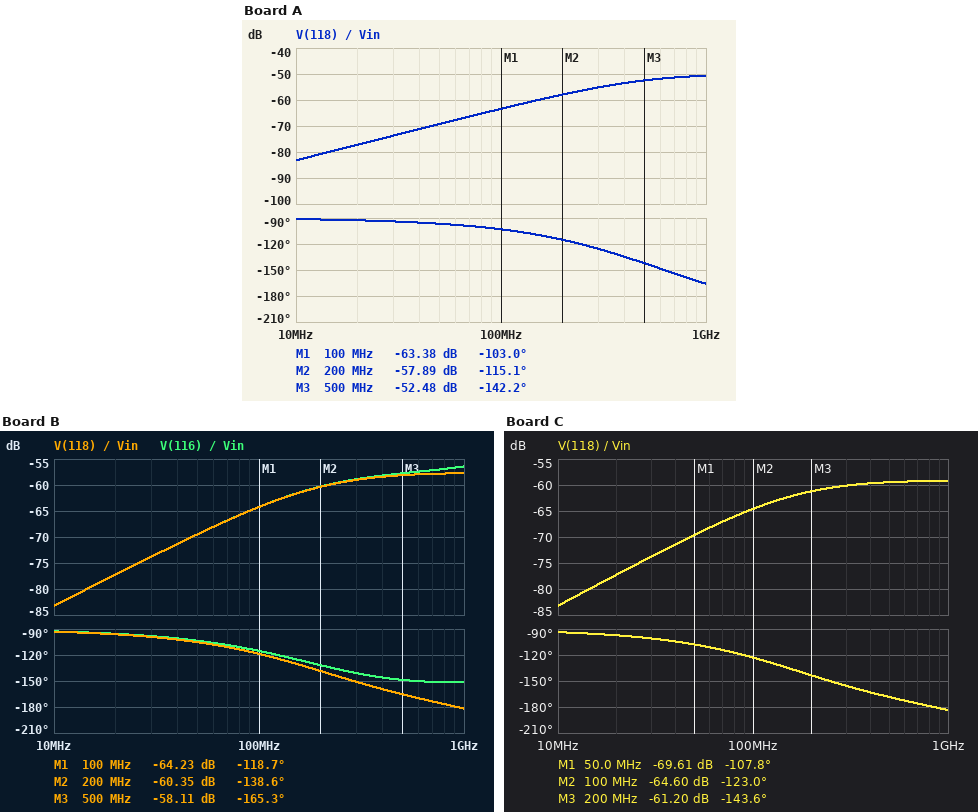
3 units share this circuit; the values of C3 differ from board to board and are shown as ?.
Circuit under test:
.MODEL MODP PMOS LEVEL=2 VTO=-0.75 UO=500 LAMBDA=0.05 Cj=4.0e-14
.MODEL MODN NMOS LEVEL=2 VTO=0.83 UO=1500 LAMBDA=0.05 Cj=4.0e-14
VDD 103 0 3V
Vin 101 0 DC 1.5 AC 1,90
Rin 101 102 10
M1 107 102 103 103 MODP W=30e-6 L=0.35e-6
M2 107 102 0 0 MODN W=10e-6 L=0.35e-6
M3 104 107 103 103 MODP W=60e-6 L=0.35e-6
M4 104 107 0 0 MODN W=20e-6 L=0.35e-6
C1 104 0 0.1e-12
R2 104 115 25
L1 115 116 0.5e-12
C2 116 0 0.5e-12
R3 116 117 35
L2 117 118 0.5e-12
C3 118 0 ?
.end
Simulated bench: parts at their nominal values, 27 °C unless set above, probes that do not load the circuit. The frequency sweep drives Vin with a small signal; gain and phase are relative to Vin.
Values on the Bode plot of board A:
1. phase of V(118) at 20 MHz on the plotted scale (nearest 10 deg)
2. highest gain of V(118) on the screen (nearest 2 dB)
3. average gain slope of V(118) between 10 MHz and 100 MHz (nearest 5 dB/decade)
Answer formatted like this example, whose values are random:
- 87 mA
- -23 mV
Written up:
- -90 deg
- -50 dB
- 20 dB/decade
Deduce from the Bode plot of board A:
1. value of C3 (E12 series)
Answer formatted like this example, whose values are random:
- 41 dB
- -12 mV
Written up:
- 820 fF
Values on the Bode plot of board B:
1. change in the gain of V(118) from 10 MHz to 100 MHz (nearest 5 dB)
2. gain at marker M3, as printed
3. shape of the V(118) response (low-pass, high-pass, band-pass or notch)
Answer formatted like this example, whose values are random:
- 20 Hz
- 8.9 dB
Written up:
- 20 dB
- -58.11 dB
- high-pass
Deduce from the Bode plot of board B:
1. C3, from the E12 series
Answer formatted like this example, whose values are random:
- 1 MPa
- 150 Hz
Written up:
- 2.7 pF
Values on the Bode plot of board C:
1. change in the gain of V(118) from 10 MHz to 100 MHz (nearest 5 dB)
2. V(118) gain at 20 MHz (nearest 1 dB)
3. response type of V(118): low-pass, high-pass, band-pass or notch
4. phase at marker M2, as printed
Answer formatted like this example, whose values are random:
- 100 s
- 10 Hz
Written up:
- 20 dB
- -77 dB
- high-pass
- -123.0 deg
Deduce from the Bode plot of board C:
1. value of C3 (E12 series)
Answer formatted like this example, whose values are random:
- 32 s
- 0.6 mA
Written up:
- 3.3 pF
